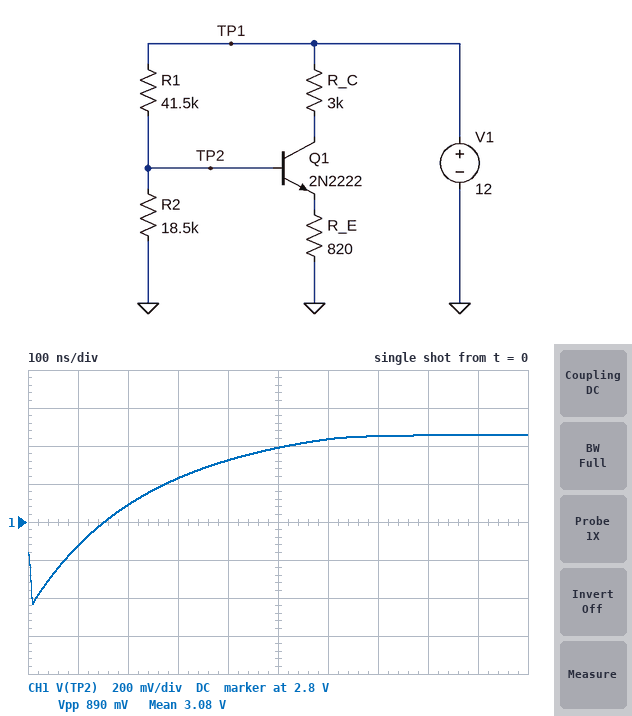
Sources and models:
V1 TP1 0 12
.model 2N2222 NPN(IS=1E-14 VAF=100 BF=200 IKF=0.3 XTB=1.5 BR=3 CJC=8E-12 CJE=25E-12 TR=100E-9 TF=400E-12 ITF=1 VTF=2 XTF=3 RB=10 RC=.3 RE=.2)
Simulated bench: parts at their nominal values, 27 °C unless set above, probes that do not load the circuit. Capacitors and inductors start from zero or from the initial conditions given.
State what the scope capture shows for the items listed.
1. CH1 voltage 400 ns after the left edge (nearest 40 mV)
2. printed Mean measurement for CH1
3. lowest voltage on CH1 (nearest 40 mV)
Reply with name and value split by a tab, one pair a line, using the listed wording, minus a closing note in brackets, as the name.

CH1 voltage 400 ns after the left edge	3.12 V
printed Mean measurement for CH1	3.08 V
lowest voltage on CH1	2.36 V
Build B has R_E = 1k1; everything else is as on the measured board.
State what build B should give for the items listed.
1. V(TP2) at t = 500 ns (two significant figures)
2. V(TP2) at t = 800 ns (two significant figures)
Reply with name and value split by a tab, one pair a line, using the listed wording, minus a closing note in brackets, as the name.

V(TP2) at t = 500 ns	3.4 V
V(TP2) at t = 800 ns	3.5 V
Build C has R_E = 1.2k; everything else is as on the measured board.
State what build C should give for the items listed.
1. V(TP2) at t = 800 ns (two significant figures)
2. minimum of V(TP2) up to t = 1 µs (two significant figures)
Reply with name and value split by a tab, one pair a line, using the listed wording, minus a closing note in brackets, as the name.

V(TP2) at t = 800 ns	3.5 V
minimum of V(TP2) up to t = 1 µs	2.9 V
